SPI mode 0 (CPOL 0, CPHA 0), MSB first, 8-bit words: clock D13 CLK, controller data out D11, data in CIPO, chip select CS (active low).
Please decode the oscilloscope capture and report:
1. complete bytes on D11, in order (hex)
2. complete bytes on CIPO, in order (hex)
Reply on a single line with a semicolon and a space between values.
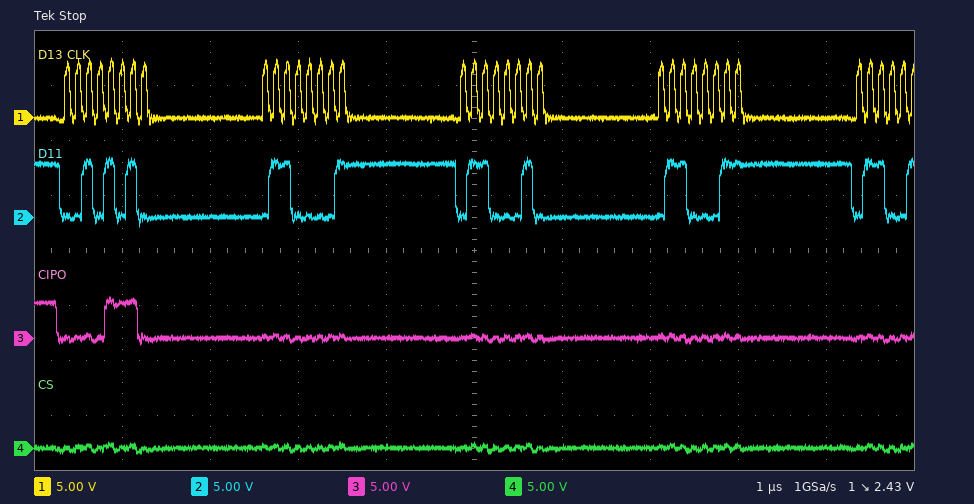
2A 61 62 63; 0E 00 00 00
